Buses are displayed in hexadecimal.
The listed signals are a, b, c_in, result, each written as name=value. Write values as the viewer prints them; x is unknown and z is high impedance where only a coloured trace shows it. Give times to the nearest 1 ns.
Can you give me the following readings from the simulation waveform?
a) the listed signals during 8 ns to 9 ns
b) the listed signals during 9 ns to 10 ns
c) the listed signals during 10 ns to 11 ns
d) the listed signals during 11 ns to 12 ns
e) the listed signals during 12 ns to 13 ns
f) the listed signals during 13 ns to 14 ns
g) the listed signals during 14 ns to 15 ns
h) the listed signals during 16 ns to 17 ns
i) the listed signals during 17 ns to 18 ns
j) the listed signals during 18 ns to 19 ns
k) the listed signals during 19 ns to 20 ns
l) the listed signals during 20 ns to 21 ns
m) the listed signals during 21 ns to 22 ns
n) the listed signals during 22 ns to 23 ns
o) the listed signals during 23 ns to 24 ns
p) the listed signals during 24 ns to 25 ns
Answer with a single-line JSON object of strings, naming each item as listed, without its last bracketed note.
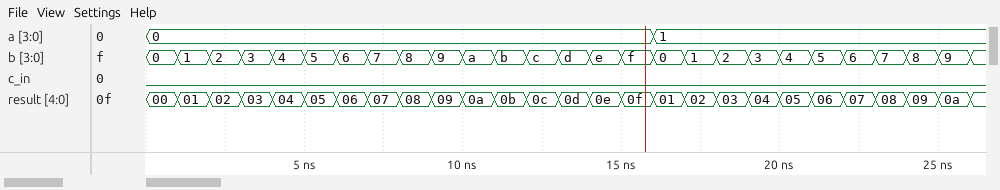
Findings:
{"the listed signals during 8 ns to 9 ns": "a=0, b=8, c_in=0, result=08", "the listed signals during 9 ns to 10 ns": "a=0, b=9, c_in=0, result=09", "the listed signals during 10 ns to 11 ns": "a=0, b=a, c_in=0, result=0a", "the listed signals during 11 ns to 12 ns": "a=0, b=b, c_in=0, result=0b", "the listed signals during 12 ns to 13 ns": "a=0, b=c, c_in=0, result=0c", "the listed signals during 13 ns to 14 ns": "a=0, b=d, c_in=0, result=0d", "the listed signals during 14 ns to 15 ns": "a=0, b=e, c_in=0, result=0e", "the listed signals during 16 ns to 17 ns": "a=1, b=0, c_in=0, result=01", "the listed signals during 17 ns to 18 ns": "a=1, b=1, c_in=0, result=02", "the listed signals during 18 ns to 19 ns": "a=1, b=2, c_in=0, result=03", "the listed signals during 19 ns to 20 ns": "a=1, b=3, c_in=0, result=04", "the listed signals during 20 ns to 21 ns": "a=1, b=4, c_in=0, result=05", "the listed signals during 21 ns to 22 ns": "a=1, b=5, c_in=0, result=06", "the listed signals during 22 ns to 23 ns": "a=1, b=6, c_in=0, result=07", "the listed signals during 23 ns to 24 ns": "a=1, b=7, c_in=0, result=08", "the listed signals during 24 ns to 25 ns": "a=1, b=8, c_in=0, result=09"}
